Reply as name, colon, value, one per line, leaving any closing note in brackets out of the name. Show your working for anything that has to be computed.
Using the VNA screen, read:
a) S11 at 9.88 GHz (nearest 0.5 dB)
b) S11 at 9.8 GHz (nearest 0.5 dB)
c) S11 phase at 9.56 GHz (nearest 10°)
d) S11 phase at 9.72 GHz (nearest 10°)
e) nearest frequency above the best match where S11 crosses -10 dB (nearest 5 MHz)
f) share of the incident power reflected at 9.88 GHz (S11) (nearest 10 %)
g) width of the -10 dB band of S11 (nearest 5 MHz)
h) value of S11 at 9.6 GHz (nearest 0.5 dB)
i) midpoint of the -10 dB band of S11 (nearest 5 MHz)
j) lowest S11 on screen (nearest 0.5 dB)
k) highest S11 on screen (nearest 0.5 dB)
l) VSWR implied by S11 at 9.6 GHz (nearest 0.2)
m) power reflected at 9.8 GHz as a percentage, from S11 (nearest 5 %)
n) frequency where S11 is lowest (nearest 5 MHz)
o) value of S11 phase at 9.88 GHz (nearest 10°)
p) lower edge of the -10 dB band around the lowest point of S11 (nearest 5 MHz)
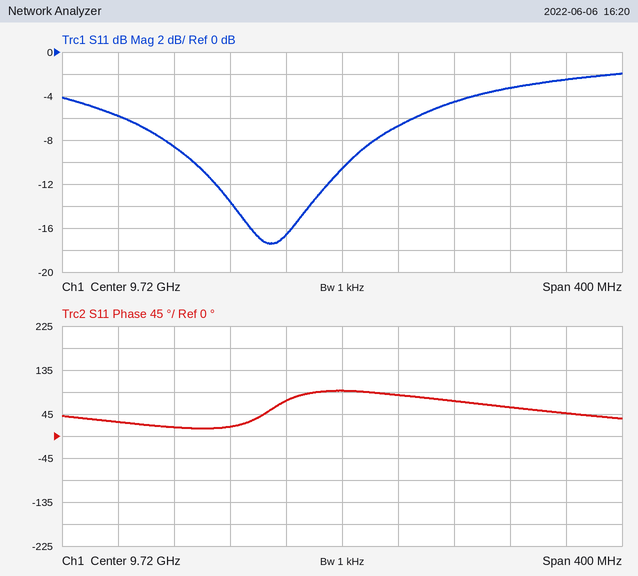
S11 at 9.88 GHz: -2.5 dB
S11 at 9.8 GHz: -4.5 dB
S11 phase at 9.56 GHz: 30°
S11 phase at 9.72 GHz: 90°
nearest frequency above the best match where S11 crosses -10 dB: 9.725 GHz
share of the incident power reflected at 9.88 GHz (S11): 10^(-2.5/10) ≈ 56.2 %, so 60 % to the nearest 10 %
width of the -10 dB band of S11: 9.725 GHz − 9.615 GHz = 110 MHz
value of S11 at 9.6 GHz: -8.5 dB
midpoint of the -10 dB band of S11: 9.670 GHz
lowest S11 on screen: -17.5 dB
highest S11 on screen: -2.0 dB
VSWR implied by S11 at 9.6 GHz: |Γ| = 10^(-8.5/20) = 0.3758; VSWR = (1 + 0.3758)/(1 − 0.3758) ≈ 2.2
power reflected at 9.8 GHz as a percentage, from S11: 10^(-4.5/10) ≈ 35 %
frequency where S11 is lowest: 9.670 GHz
value of S11 phase at 9.88 GHz: 50°
lower edge of the -10 dB band around the lowest point of S11: 9.615 GHz
